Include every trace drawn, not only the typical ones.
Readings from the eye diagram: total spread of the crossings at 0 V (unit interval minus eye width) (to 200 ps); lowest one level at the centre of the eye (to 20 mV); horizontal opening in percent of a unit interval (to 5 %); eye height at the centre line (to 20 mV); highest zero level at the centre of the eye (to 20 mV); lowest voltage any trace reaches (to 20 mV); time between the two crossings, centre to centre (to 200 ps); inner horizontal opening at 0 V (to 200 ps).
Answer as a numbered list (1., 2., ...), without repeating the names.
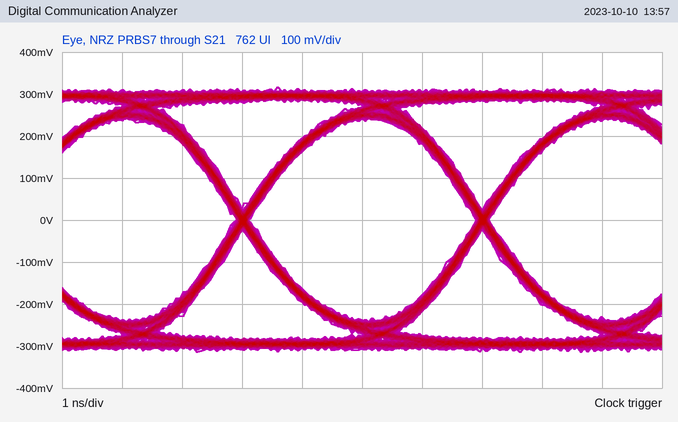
1. 200 ps
2. 240 mV
3. 95 %
4. 480 mV
5. -240 mV
6. -320 mV
7. 4.0 ns
8. 3.8 ns
